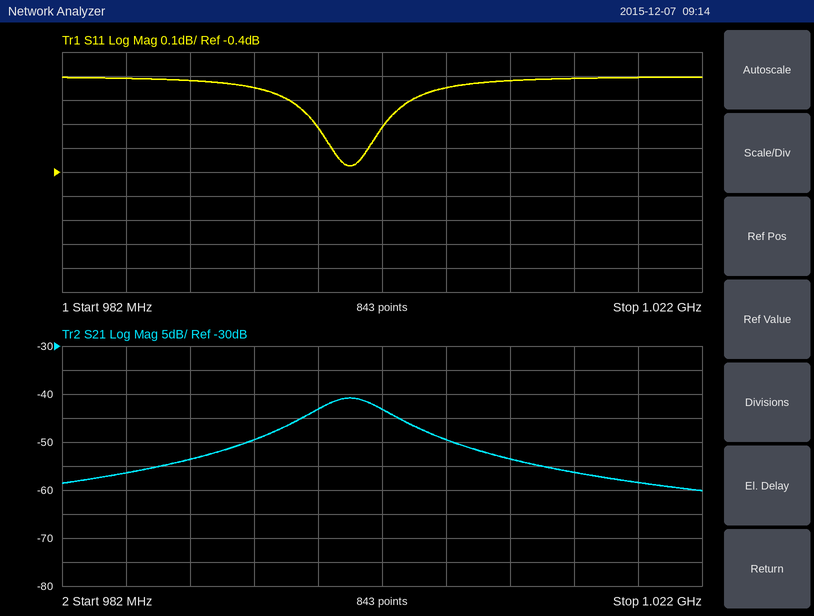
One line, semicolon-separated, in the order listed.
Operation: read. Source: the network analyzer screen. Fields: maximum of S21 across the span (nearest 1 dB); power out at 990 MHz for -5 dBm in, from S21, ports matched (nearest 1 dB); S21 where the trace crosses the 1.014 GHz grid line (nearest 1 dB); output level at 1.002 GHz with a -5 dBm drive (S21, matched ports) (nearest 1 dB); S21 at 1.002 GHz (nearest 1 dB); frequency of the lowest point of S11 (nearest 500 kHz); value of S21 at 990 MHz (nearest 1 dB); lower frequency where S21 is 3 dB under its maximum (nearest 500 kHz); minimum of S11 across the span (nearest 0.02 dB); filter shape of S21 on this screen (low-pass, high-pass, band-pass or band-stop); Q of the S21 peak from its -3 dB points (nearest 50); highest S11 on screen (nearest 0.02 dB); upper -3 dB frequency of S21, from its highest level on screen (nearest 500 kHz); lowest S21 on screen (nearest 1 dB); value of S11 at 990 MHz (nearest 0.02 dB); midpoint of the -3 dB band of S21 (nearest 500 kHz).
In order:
-41 dB; -59 dBm; -56 dB; -48 dBm; -43 dB; 1.0000 GHz; -54 dB; 997.5 MHz; -0.38 dB; band-pass; 200; 0.00 dB; 1.0025 GHz; -60 dB; -0.02 dB; 1.0000 GHz
